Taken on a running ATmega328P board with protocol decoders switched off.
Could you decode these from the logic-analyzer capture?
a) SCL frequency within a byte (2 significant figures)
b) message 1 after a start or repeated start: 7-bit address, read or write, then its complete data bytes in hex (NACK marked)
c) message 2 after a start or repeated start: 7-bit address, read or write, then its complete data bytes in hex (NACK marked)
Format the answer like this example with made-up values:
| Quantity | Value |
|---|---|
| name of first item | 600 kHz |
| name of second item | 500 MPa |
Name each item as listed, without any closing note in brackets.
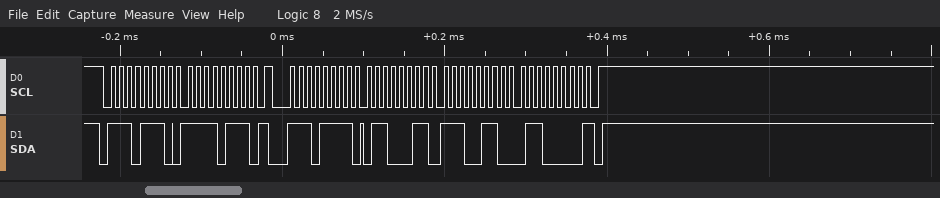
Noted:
| Quantity | Value |
|---|---|
| SCL frequency within a byte | 100 kHz |
| message 1 after a start or repeated start: 7-bit address, read or write, then its complete data bytes in hex | 0x77 write: F7 |
| message 2 after a start or repeated start: 7-bit address, read or write, then its complete data bytes in hex | 0x77 read: 63 E6 60 NACK |
